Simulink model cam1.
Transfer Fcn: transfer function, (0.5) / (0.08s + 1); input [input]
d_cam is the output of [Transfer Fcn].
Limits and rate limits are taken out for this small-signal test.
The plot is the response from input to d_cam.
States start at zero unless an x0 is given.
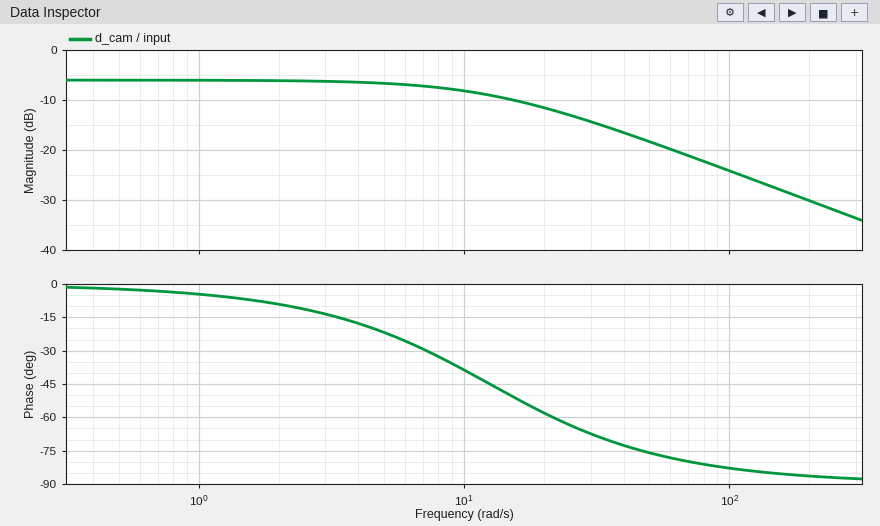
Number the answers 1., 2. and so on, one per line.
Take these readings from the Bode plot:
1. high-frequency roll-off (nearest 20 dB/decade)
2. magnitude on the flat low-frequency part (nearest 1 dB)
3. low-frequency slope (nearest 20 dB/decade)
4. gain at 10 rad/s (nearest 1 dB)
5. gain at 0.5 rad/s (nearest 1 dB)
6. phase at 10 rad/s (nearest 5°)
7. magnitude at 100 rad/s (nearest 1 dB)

1. -20 dB/decade
2. -6 dB
3. 0 dB/decade
4. -8 dB
5. -6 dB
6. -40°
7. -24 dB
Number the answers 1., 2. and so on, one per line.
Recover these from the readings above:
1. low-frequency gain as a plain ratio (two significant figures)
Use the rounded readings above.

1. 0.50
